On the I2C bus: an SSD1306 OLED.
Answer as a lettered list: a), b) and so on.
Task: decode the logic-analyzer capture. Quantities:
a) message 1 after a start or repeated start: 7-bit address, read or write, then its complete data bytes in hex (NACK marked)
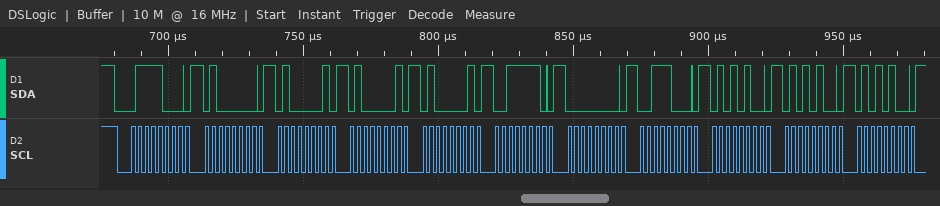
a) 0x3C write: 40 41 41 41 3E 00 38 54 54 54
